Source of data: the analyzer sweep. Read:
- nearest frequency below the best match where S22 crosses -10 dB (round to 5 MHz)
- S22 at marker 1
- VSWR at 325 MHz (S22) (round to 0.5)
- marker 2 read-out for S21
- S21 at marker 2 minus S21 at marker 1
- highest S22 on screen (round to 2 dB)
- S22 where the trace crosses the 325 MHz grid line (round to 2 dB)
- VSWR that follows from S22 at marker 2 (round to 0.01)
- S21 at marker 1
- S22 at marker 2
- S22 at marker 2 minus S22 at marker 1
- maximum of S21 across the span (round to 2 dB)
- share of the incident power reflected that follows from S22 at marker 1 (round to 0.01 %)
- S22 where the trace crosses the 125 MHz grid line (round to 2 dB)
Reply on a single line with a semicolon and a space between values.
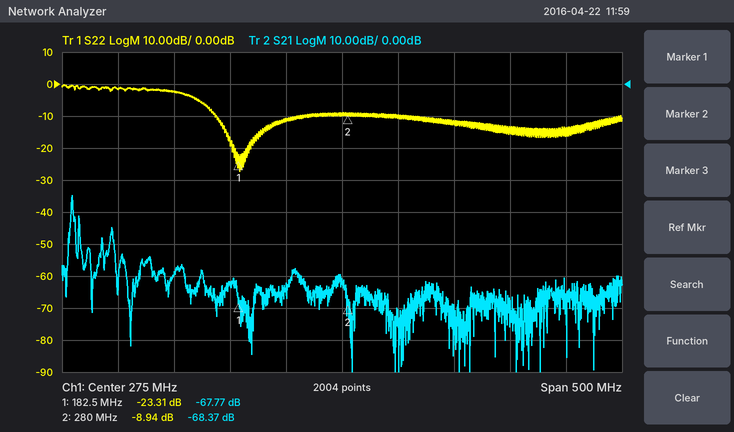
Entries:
165 MHz; -23.31 dB; 2.0; -68.37 dB; -0.60 dB; 0 dB; -10 dB; 2.11; -67.77 dB; -8.94 dB; 14.37 dB; -34 dB; 0.47 %; -2 dB
